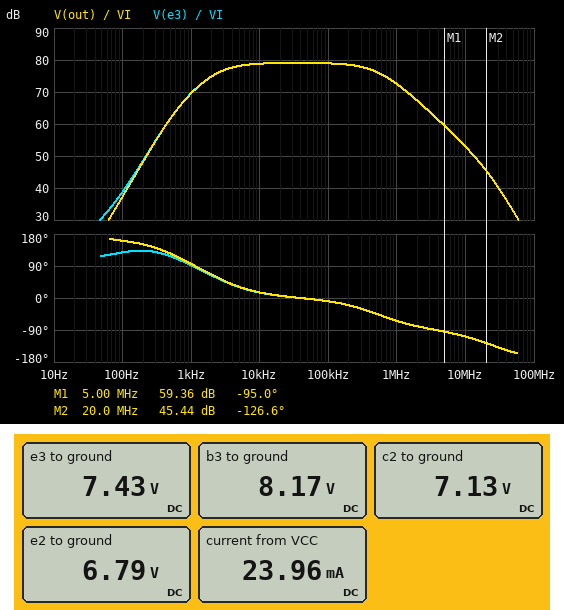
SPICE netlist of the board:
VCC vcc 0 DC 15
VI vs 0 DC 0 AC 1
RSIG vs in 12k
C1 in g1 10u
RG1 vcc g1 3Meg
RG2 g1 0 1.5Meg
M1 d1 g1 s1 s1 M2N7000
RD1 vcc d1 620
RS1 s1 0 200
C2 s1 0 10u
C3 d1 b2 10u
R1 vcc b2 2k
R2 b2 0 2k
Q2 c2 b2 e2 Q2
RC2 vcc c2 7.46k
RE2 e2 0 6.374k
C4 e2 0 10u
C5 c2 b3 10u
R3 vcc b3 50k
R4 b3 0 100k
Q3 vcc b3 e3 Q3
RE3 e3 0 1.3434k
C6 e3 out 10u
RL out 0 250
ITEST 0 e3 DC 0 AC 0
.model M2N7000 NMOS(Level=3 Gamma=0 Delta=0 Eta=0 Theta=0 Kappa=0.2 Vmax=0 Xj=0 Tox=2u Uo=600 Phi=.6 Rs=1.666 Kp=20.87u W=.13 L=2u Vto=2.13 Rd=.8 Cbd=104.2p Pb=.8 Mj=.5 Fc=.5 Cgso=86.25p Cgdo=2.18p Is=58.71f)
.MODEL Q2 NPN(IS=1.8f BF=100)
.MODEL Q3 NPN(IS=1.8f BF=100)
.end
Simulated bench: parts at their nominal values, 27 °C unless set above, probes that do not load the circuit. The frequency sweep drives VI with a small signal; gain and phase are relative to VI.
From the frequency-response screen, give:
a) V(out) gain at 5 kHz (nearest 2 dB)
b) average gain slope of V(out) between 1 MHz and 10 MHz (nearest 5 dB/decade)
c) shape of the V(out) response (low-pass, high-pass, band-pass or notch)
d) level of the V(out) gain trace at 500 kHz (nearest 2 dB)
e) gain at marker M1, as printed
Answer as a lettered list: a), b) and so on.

a) 78 dB
b) -20 dB/decade
c) band-pass
d) 76 dB
e) 59.36 dB
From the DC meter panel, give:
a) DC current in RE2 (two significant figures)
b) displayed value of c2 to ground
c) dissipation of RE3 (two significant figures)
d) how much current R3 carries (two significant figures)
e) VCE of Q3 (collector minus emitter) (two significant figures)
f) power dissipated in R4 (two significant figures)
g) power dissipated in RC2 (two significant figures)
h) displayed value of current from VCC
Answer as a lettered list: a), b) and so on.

a) 1.1 mA
b) 7.13 V
c) 41 mW
d) 140 µA
e) 7.6 V
f) 670 µW
g) 8.3 mW
h) 23.96 mA
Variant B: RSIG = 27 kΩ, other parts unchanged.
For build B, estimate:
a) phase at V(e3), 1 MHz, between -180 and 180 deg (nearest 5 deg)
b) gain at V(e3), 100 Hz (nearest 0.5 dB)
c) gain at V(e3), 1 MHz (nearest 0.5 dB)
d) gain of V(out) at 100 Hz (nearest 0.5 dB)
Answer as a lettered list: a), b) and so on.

a) -80 deg
b) 38.5 dB
c) 66.5 dB
d) 37.0 dB
